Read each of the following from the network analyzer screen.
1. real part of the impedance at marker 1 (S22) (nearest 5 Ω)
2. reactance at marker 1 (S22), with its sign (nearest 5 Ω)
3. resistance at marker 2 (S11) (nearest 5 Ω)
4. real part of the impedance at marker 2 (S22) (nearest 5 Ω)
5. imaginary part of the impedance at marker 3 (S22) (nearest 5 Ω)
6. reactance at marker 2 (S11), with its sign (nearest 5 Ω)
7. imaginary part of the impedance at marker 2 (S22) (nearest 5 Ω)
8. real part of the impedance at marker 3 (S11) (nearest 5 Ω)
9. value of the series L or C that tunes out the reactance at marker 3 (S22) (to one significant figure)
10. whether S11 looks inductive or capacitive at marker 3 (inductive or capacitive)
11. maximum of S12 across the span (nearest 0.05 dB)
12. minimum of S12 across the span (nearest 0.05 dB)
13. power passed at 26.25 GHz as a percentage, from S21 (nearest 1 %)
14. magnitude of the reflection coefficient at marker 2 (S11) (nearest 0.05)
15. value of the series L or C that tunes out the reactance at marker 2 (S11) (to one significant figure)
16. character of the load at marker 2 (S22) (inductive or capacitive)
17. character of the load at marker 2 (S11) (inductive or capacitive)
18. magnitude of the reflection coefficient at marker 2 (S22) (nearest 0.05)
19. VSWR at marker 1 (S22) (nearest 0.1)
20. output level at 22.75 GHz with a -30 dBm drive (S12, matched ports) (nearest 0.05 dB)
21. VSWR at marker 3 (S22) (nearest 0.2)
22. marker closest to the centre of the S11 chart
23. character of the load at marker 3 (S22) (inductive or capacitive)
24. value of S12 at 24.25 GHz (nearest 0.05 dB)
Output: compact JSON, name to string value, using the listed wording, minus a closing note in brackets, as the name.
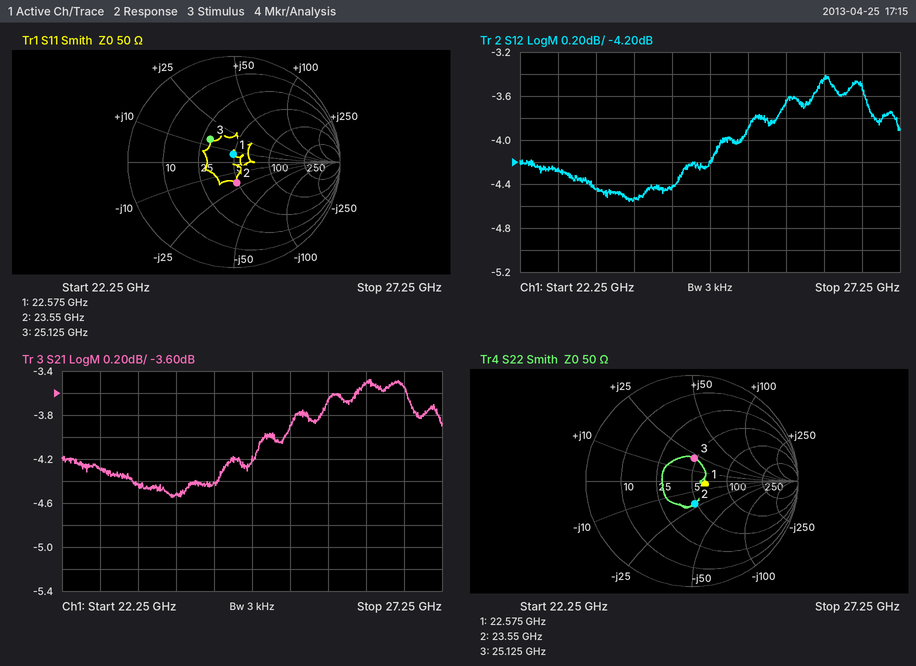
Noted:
{"real part of the impedance at marker 1 (S22)": "65 Ω", "reactance at marker 1 (S22), with its sign": "-5 Ω", "resistance at marker 2 (S11)": "50 Ω", "real part of the impedance at marker 2 (S22)": "50 Ω", "imaginary part of the impedance at marker 3 (S22)": "+20 Ω", "reactance at marker 2 (S11), with its sign": "-20 Ω", "imaginary part of the impedance at marker 2 (S22)": "-20 Ω", "real part of the impedance at marker 3 (S11)": "30 Ω", "value of the series L or C that tunes out the reactance at marker 3 (S22)": "300 fF", "whether S11 looks inductive or capacitive at marker 3": "inductive", "maximum of S12 across the span": "-3.40 dB", "minimum of S12 across the span": "-4.55 dB", "power passed at 26.25 GHz as a percentage, from S21": "45 %", "magnitude of the reflection coefficient at marker 2 (S11)": "0.20", "value of the series L or C that tunes out the reactance at marker 2 (S11)": "100 pH", "character of the load at marker 2 (S22)": "capacitive", "character of the load at marker 2 (S11)": "capacitive", "magnitude of the reflection coefficient at marker 2 (S22)": "0.20", "VSWR at marker 1 (S22)": "1.3", "output level at 22.75 GHz with a -30 dBm drive (S12, matched ports)": "-34.25 dBm", "VSWR at marker 3 (S22)": "1.6", "marker closest to the centre of the S11 chart": "marker 1", "character of the load at marker 3 (S22)": "inductive", "value of S12 at 24.25 GHz": "-4.45 dB"}
